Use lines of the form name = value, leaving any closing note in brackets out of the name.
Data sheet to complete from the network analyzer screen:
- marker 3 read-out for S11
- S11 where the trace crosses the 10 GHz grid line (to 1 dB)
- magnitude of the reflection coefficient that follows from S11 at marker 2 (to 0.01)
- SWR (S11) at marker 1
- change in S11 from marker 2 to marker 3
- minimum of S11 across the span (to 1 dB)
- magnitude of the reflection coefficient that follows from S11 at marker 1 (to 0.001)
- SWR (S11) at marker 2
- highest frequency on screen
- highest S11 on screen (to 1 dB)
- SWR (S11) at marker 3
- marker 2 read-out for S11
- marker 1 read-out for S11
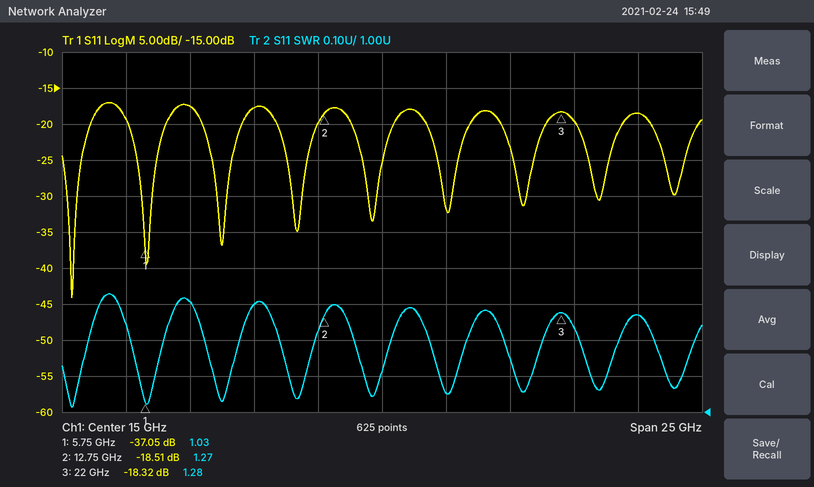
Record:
marker 3 read-out for S11 = -18.32 dB
S11 where the trace crosses the 10 GHz grid line = -18 dB
magnitude of the reflection coefficient that follows from S11 at marker 2 = 0.12
SWR (S11) at marker 1 = 1.03
change in S11 from marker 2 to marker 3 = 0.19 dB
minimum of S11 across the span = -44 dB
magnitude of the reflection coefficient that follows from S11 at marker 1 = 0.014
SWR (S11) at marker 2 = 1.27
highest frequency on screen = 27.5 GHz
highest S11 on screen = -17 dB
SWR (S11) at marker 3 = 1.28
marker 2 read-out for S11 = -18.51 dB
marker 1 read-out for S11 = -37.05 dB
